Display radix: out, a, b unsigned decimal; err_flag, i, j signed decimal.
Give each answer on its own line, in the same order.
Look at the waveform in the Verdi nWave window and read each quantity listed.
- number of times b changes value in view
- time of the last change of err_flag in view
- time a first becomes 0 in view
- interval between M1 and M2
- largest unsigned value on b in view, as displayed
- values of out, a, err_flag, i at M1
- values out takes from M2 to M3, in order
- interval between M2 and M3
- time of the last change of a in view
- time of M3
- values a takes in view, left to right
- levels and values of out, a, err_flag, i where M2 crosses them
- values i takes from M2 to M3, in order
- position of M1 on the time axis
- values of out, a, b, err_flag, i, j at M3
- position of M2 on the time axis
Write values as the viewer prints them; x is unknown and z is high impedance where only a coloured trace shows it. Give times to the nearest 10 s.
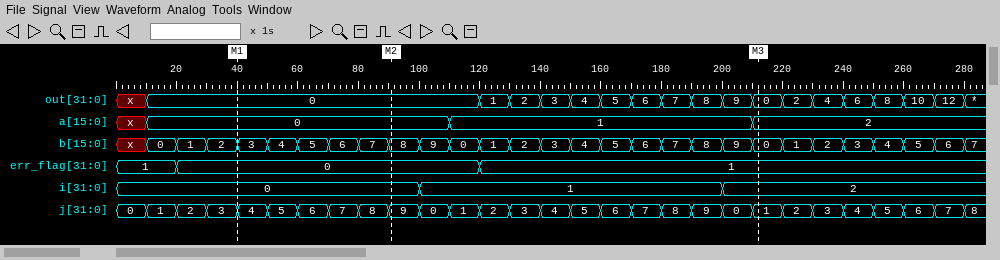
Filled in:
28
120 s
10 s
50 s
9
out=0, a=0, err_flag=0, i=0
0, 1, 2, 3, 4, 5, 6, 7, 8, 9, 0
120 s
210 s
210 s
x, 0, 1, 2
out=0, a=0, err_flag=0, i=0
0, 1, 2
40 s
out=0, a=2, b=0, err_flag=1, i=2, j=1
90 s
